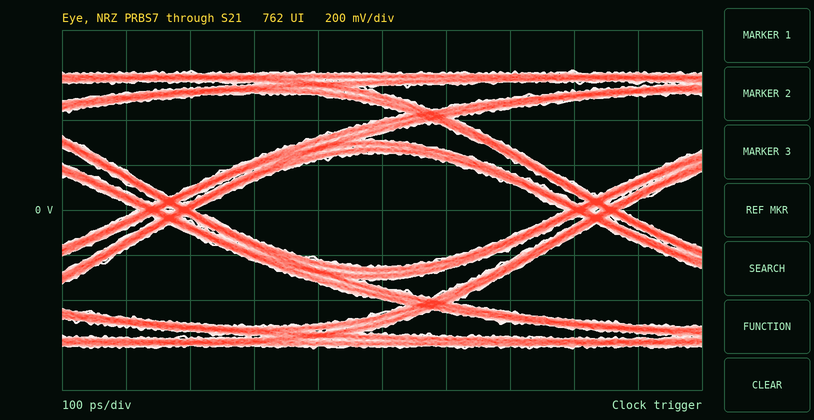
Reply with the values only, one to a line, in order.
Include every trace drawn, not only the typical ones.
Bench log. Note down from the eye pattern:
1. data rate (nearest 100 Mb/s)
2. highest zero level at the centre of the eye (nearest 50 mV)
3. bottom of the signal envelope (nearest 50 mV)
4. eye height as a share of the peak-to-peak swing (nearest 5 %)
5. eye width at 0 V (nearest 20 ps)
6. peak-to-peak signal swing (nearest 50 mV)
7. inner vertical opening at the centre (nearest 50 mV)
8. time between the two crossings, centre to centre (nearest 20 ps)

1.5 Gb/s
-250 mV
-600 mV
40 %
580 ps
1.25 V
500 mV
660 ps
